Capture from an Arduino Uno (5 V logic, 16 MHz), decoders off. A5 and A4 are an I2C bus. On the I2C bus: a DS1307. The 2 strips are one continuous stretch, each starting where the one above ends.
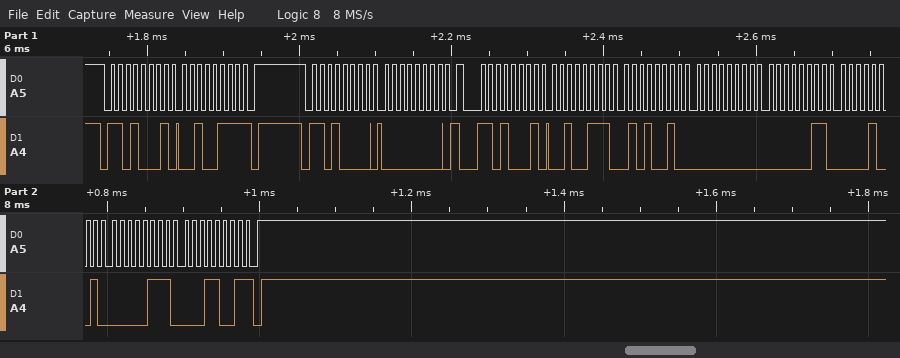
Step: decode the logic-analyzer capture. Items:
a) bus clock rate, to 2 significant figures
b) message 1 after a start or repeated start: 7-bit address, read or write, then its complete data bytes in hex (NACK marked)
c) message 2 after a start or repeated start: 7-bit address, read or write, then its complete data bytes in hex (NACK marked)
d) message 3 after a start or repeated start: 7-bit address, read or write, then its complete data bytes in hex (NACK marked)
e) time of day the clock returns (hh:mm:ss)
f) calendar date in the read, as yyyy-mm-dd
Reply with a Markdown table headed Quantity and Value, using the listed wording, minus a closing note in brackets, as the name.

| Quantity | Value |
|---|---|
| bus clock rate, to 2 significant figures | 100 kHz |
| message 1 after a start or repeated start: 7-bit address, read or write, then its complete data bytes in hex | 0x68 read: 27 NACK |
| message 2 after a start or repeated start: 7-bit address, read or write, then its complete data bytes in hex | 0x68 write: 00 |
| message 3 after a start or repeated start: 7-bit address, read or write, then its complete data bytes in hex | 0x68 read: 27 52 00 03 09 07 19 NACK |
| time of day the clock returns | 00:52:27 |
| calendar date in the read, as yyyy-mm-dd | 2019-07-09 |
